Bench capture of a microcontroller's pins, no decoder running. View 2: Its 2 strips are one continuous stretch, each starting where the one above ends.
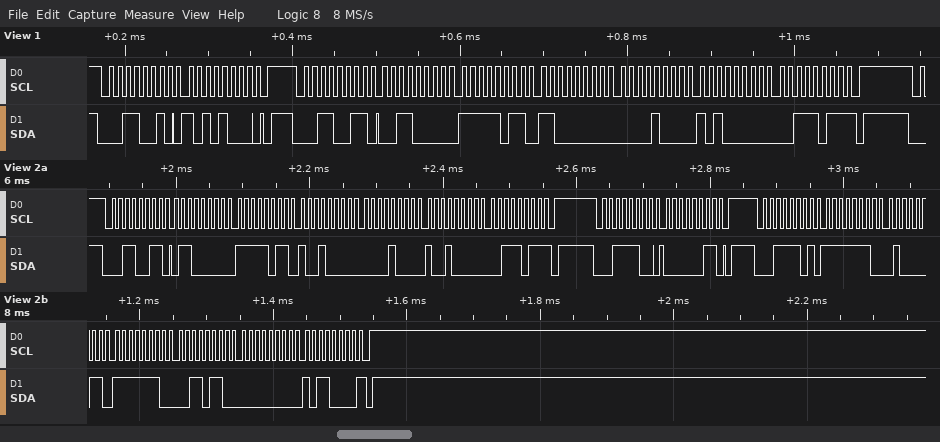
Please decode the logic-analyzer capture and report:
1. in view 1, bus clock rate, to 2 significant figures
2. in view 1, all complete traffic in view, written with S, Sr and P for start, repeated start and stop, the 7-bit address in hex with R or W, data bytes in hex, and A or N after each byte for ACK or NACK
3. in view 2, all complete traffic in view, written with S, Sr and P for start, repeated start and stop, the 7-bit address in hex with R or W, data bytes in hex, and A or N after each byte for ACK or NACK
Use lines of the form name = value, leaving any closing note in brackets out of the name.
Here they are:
in view 1, bus clock rate, to 2 significant figures = 100 kHz
in view 1, all complete traffic in view, written with S, Sr and P for start, repeated start and stop, the 7-bit address in hex with R or W, data bytes in hex, and A or N after each byte for ACK or NACK = S 19W A A8 A P S 19R A 30 A FB A C0 A 08 A A0 A 3B N P
in view 2, all complete traffic in view, written with S, Sr and P for start, repeated start and stop, the 7-bit address in hex with R or W, data bytes in hex, and A or N after each byte for ACK or NACK = S 19R A 60 A FB A 90 A 08 A 90 A 3B N P S 1EW A 03 A P S 1ER A FE A 43 A FE A 36 A 00 A B0 N P
